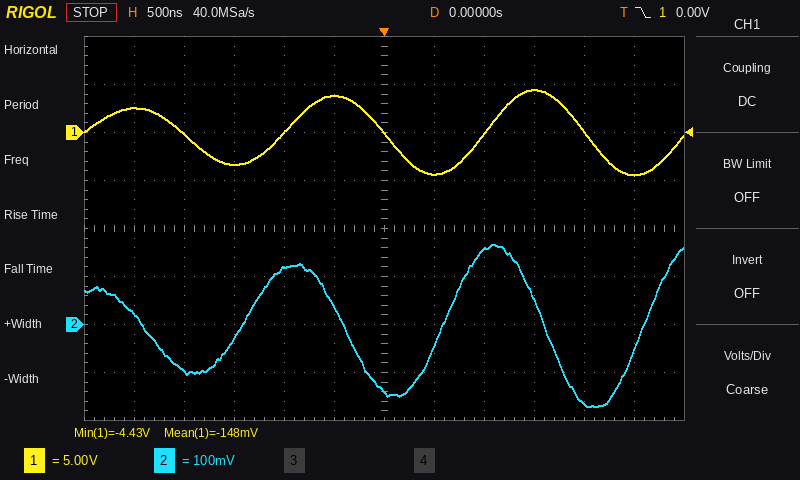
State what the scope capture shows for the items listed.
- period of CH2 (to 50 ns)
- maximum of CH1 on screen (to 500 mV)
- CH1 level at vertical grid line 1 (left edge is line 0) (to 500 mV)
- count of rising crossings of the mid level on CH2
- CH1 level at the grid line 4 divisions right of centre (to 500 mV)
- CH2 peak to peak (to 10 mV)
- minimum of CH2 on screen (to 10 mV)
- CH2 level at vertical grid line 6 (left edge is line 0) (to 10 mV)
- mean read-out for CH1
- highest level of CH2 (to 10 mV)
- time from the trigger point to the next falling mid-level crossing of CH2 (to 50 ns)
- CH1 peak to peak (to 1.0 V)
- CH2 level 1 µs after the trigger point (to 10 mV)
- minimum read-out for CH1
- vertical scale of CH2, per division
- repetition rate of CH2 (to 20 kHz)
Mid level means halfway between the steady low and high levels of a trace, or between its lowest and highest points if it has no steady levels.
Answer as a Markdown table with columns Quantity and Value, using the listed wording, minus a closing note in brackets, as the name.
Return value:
| Quantity | Value |
|---|---|
| period of CH2 | 2.00 µs |
| maximum of CH1 on screen | 4.5 V |
| CH1 level at vertical grid line 1 (left edge is line 0) | 2.5 V |
| count of rising crossings of the mid level on CH2 | 3 |
| CH1 level at the grid line 4 divisions right of centre | 0.0 V |
| CH2 peak to peak | 340 mV |
| minimum of CH2 on screen | -170 mV |
| CH2 level at vertical grid line 6 (left edge is line 0) | -140 mV |
| mean read-out for CH1 | -148 mV |
| highest level of CH2 | 170 mV |
| time from the trigger point to the next falling mid-level crossing of CH2 | 1.60 µs |
| CH1 peak to peak | 9.0 V |
| CH2 level 1 µs after the trigger point | 160 mV |
| minimum read-out for CH1 | -4.43 V |
| vertical scale of CH2, per division | 100 mV |
| repetition rate of CH2 | 500 kHz |
